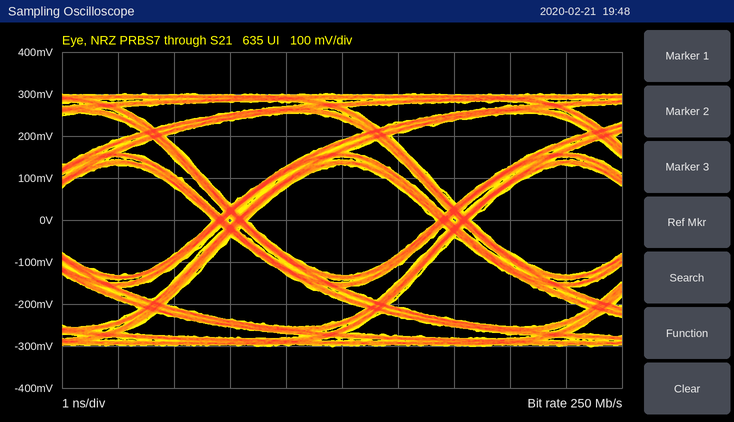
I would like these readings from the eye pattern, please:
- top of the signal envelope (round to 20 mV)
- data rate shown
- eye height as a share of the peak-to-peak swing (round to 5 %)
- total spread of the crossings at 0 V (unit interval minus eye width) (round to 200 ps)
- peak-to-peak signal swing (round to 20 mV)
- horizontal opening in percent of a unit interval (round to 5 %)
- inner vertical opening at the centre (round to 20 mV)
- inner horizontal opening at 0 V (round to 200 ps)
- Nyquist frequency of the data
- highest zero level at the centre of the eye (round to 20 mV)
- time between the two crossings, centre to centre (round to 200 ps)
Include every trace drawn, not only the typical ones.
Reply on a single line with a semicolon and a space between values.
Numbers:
300 mV; 250 Mb/s; 45 %; 600 ps; 600 mV; 85 %; 260 mV; 3.4 ns; 125 MHz; -140 mV; 4.0 ns
